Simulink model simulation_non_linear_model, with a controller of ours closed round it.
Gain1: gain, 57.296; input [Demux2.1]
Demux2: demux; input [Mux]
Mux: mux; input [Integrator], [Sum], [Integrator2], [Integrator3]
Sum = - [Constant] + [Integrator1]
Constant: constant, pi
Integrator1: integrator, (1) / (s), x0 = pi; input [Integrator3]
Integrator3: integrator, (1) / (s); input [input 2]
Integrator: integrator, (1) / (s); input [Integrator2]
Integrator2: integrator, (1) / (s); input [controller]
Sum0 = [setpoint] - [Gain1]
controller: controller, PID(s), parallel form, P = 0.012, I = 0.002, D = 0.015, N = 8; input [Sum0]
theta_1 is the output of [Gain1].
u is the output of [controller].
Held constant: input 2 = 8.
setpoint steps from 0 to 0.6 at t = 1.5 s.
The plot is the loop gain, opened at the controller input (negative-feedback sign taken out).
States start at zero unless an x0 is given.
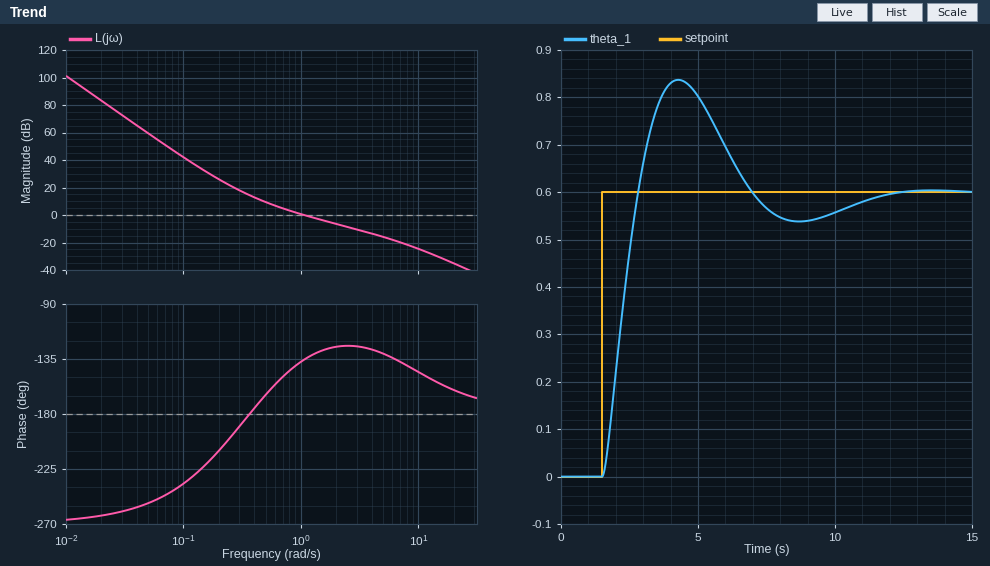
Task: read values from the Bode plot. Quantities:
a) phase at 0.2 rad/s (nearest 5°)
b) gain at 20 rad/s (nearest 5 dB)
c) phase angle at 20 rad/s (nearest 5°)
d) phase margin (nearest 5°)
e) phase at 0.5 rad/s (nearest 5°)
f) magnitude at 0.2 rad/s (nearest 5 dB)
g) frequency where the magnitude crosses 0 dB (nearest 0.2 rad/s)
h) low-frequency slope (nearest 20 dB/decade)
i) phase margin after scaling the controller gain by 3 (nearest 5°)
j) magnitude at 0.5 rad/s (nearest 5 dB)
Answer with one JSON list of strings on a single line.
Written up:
["-210°", "-35 dB", "-160°", "45°", "-165°", "25 dB", "1.0 rad/s", "-60 dB/decade", "55°", "10 dB"]
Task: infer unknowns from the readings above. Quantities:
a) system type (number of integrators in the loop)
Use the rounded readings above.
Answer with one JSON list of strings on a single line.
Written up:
["3"]
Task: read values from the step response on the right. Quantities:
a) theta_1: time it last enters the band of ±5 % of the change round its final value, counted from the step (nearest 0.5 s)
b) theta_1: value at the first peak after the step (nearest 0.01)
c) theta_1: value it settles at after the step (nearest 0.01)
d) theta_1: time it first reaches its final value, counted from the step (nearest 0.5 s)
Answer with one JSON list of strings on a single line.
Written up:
["9.0 s", "0.84", "0.60", "1.5 s"]
